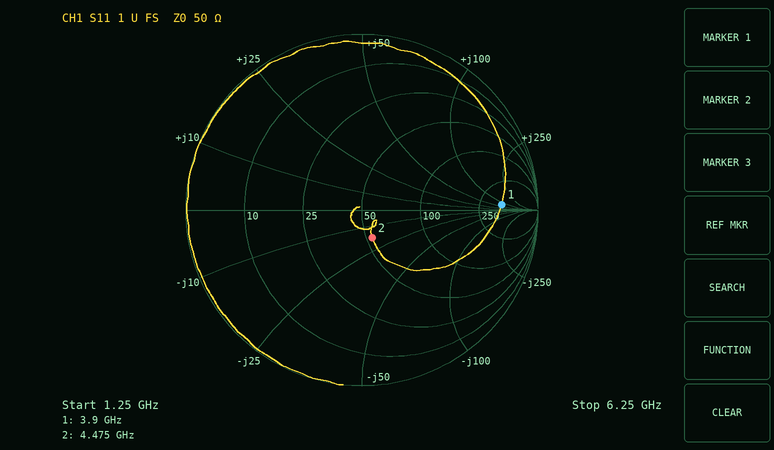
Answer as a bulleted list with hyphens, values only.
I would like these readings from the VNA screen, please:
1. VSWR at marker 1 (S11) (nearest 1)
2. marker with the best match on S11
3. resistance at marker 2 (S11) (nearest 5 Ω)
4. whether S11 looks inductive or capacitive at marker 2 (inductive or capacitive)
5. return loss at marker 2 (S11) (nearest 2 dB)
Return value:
- 9
- marker 2
- 55 Ω
- capacitive
- 16 dB
